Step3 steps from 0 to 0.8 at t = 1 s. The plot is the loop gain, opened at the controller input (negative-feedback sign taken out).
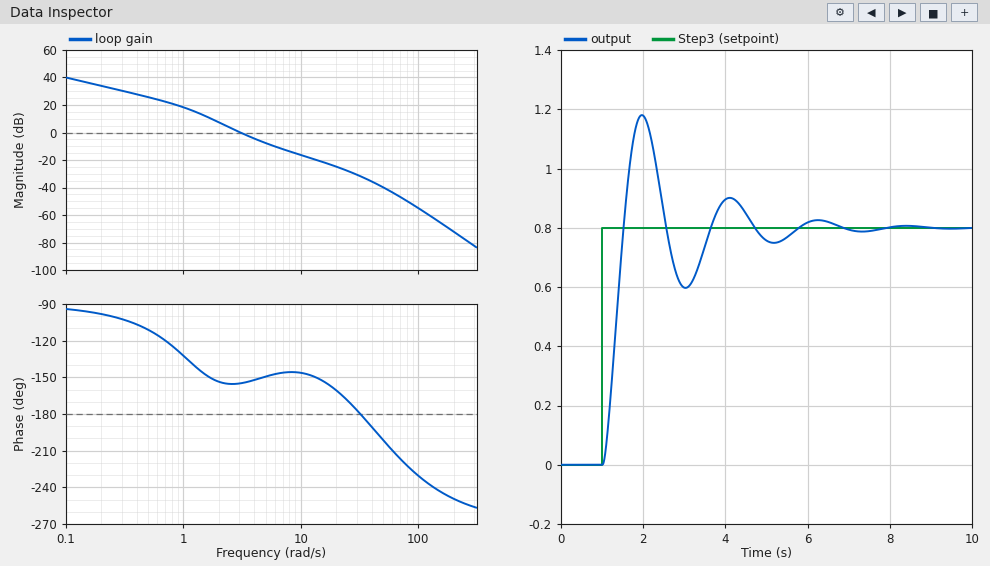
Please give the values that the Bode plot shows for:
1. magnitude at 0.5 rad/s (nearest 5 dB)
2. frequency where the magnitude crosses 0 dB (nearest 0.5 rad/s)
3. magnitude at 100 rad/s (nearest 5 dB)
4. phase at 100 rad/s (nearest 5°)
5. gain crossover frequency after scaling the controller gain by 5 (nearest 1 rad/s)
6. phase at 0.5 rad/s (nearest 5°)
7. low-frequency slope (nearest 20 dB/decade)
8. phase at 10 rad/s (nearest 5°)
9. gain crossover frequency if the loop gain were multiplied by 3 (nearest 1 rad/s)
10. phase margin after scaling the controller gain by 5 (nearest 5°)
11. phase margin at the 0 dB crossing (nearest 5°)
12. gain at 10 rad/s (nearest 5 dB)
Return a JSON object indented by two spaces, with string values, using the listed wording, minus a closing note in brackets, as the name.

{
  "magnitude at 0.5 rad/s": "25 dB",
  "frequency where the magnitude crosses 0 dB": "3.0 rad/s",
  "magnitude at 100 rad/s": "-55 dB",
  "phase at 100 rad/s": "-230°",
  "gain crossover frequency after scaling the controller gain by 5": "8 rad/s",
  "phase at 0.5 rad/s": "-110°",
  "low-frequency slope": "-20 dB/decade",
  "phase at 10 rad/s": "-145°",
  "gain crossover frequency if the loop gain were multiplied by 3": "6 rad/s",
  "phase margin after scaling the controller gain by 5": "35°",
  "phase margin at the 0 dB crossing": "25°",
  "gain at 10 rad/s": "-15 dB"
}
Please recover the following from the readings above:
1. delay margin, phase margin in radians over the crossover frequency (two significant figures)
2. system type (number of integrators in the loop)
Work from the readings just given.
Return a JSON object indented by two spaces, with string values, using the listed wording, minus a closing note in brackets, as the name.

{
  "delay margin, phase margin in radians over the crossover frequency": "0.15 s",
  "system type": "1"
}
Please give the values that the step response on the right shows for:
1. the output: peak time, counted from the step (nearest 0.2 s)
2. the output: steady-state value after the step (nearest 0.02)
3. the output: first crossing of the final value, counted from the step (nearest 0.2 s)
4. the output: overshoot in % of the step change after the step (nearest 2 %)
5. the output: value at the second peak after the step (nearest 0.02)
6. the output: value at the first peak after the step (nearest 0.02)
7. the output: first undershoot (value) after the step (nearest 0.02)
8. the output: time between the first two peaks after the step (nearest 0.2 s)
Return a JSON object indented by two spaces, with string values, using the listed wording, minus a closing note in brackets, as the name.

{
  "the output: peak time, counted from the step": "1.0 s",
  "the output: steady-state value after the step": "0.80",
  "the output: first crossing of the final value, counted from the step": "0.6 s",
  "the output: overshoot in % of the step change after the step": "48 %",
  "the output: value at the second peak after the step": "0.90",
  "the output: value at the first peak after the step": "1.18",
  "the output: first undershoot (value) after the step": "0.60",
  "the output: time between the first two peaks after the step": "2.2 s"
}
